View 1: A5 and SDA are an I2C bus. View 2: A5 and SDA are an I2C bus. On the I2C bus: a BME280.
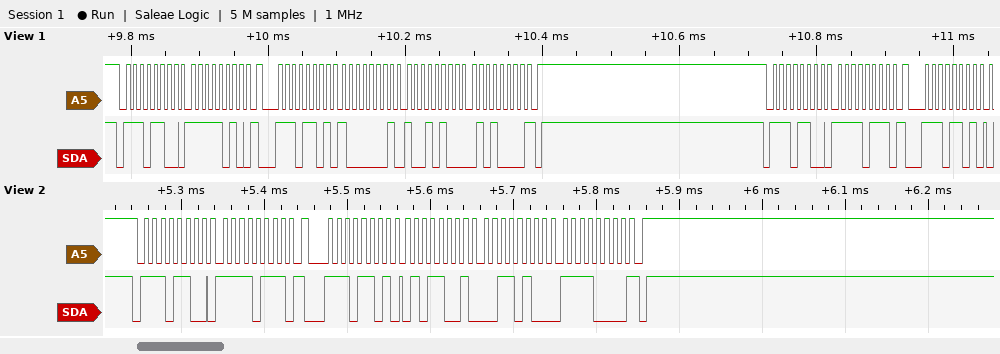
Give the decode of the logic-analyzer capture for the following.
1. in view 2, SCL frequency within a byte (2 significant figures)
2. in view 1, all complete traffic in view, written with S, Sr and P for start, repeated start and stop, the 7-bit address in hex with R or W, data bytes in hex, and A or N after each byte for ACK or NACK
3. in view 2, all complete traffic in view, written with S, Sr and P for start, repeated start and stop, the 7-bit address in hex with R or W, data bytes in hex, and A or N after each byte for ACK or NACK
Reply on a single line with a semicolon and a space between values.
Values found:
100 kHz; S 76W A FA A Sr 76R A 81 A 94 A 50 N P S 76W A F7 A Sr 76R A; S 76W A F7 A Sr 76R A 59 A 34 A F0 N P
